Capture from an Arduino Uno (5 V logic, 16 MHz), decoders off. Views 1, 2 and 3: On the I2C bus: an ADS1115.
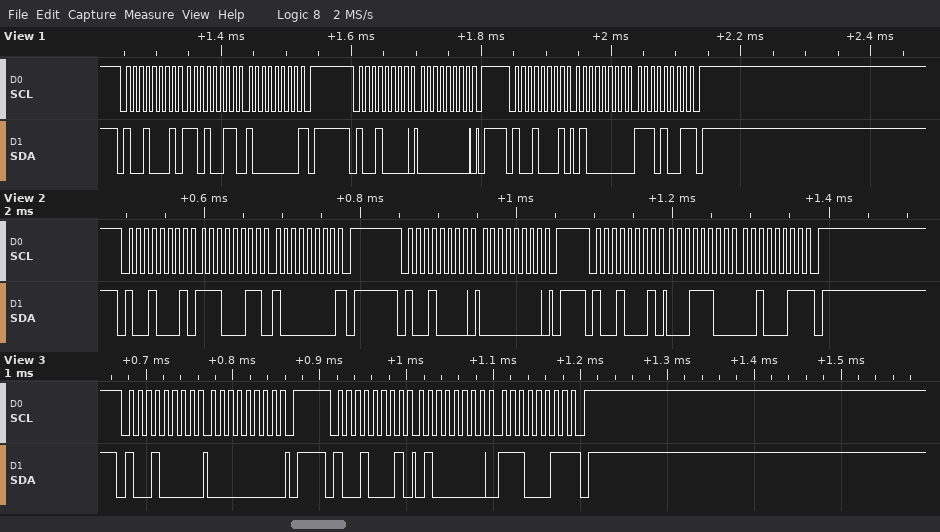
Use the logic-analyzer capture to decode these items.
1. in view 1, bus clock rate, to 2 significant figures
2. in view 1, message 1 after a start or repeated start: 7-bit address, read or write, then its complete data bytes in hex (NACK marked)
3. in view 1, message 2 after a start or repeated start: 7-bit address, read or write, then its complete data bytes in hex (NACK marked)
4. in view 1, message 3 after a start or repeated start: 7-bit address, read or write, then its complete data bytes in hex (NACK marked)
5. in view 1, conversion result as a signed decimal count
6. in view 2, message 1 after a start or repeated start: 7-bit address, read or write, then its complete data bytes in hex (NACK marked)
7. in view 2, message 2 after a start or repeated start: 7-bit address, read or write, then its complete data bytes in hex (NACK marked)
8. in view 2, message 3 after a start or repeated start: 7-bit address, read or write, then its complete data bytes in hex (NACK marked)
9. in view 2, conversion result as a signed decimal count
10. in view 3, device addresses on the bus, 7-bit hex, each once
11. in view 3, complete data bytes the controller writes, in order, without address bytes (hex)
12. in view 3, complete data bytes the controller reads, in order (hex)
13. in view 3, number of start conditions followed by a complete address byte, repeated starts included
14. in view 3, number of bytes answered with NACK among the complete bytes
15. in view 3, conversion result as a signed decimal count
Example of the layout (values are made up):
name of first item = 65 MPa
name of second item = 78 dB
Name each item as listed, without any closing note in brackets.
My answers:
in view 1, bus clock rate, to 2 significant figures = 100 kHz
in view 1, message 1 after a start or repeated start: 7-bit address, read or write, then its complete data bytes in hex = 0x48 read: D3 80 NACK
in view 1, message 2 after a start or repeated start: 7-bit address, read or write, then its complete data bytes in hex = 0x48 write: 00
in view 1, message 3 after a start or repeated start: 7-bit address, read or write, then its complete data bytes in hex = 0x48 read: 40 E9 NACK
in view 1, conversion result as a signed decimal count = 16617
in view 2, message 1 after a start or repeated start: 7-bit address, read or write, then its complete data bytes in hex = 0x48 read: E3 80 NACK
in view 2, message 2 after a start or repeated start: 7-bit address, read or write, then its complete data bytes in hex = 0x48 write: 00
in view 2, message 3 after a start or repeated start: 7-bit address, read or write, then its complete data bytes in hex = 0x48 read: 1C 23 NACK
in view 2, conversion result as a signed decimal count = 7203
in view 3, device addresses on the bus, 7-bit hex, each once = 0x48
in view 3, complete data bytes the controller writes, in order, without address bytes = 00
in view 3, complete data bytes the controller reads, in order = 40 E3
in view 3, number of start conditions followed by a complete address byte, repeated starts included = 2
in view 3, number of bytes answered with NACK among the complete bytes = 1
in view 3, conversion result as a signed decimal count = 16611
